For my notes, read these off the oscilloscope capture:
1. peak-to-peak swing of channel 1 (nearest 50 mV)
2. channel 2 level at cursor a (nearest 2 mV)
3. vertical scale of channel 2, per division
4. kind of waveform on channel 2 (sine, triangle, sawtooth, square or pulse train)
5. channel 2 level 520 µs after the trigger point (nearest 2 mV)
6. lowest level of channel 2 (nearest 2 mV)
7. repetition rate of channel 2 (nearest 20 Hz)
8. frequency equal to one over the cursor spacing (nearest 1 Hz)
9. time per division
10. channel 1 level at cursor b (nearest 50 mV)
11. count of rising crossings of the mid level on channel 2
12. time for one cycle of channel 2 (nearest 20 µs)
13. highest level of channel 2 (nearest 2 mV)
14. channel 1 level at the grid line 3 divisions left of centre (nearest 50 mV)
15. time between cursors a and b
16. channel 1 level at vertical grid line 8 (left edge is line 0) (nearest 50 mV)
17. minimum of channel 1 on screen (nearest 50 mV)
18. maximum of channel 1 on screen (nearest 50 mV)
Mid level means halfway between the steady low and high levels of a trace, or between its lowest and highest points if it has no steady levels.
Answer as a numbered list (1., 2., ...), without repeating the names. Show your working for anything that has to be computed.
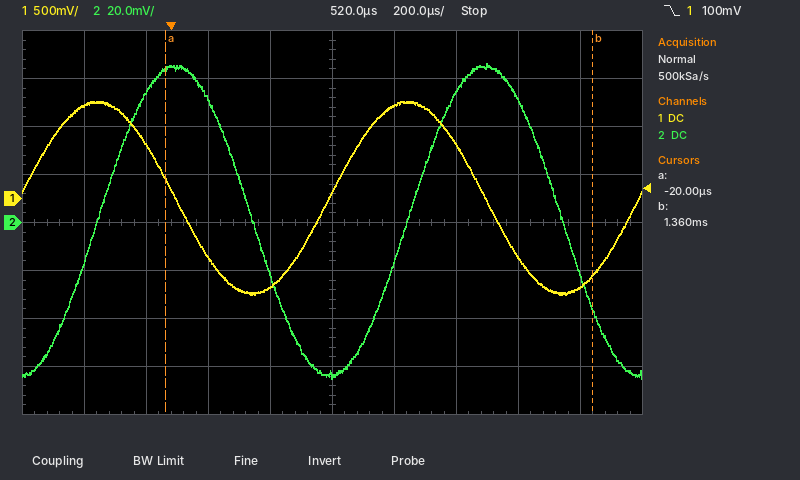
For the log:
1. 1.00 V − (-1.00 V) = 2.00 V
2. 64 mV
3. 20 mV
4. sine
5. -64 mV
6. -64 mV
7. 1 / 1.00 ms ≈ 1.00 kHz
8. 1 / 1.38 ms ≈ 725 Hz
9. 200 µs
10. -800 mV
11. 2
12. 1.00 ms
13. 66 mV
14. 550 mV
15. 1.36 ms − (-20 µs) = 1.38 ms
16. -600 mV
17. -1.00 V
18. 1.00 V
